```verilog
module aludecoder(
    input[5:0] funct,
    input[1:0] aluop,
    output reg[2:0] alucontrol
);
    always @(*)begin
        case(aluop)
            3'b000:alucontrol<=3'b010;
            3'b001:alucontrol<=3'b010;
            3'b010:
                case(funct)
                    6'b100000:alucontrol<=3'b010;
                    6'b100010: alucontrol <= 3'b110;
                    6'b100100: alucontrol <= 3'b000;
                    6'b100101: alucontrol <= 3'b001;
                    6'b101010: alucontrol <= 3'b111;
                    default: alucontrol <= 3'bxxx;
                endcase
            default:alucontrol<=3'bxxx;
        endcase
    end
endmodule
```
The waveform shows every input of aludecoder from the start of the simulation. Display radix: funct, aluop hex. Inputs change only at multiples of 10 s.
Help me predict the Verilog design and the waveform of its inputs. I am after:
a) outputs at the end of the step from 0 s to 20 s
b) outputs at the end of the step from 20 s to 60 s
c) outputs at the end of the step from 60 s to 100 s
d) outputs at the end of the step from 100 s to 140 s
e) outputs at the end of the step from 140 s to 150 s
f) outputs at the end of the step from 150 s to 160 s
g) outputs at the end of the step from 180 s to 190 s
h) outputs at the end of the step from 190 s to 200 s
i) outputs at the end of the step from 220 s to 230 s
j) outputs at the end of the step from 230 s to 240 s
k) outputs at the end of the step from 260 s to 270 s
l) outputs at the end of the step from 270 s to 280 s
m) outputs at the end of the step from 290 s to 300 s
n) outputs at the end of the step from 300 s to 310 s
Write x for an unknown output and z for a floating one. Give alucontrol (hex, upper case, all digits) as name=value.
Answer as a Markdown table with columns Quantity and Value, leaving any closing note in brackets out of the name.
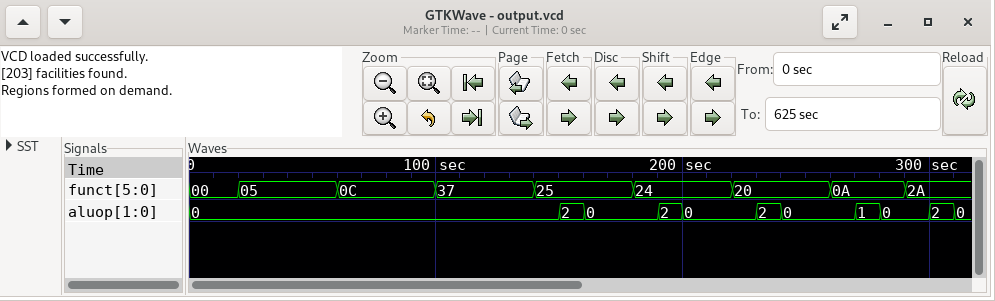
| Quantity | Value |
|---|---|
| outputs at the end of the step from 0 s to 20 s | alucontrol=2 |
| outputs at the end of the step from 20 s to 60 s | alucontrol=2 |
| outputs at the end of the step from 60 s to 100 s | alucontrol=2 |
| outputs at the end of the step from 100 s to 140 s | alucontrol=2 |
| outputs at the end of the step from 140 s to 150 s | alucontrol=2 |
| outputs at the end of the step from 150 s to 160 s | alucontrol=1 |
| outputs at the end of the step from 180 s to 190 s | alucontrol=2 |
| outputs at the end of the step from 190 s to 200 s | alucontrol=0 |
| outputs at the end of the step from 220 s to 230 s | alucontrol=2 |
| outputs at the end of the step from 230 s to 240 s | alucontrol=2 |
| outputs at the end of the step from 260 s to 270 s | alucontrol=2 |
| outputs at the end of the step from 270 s to 280 s | alucontrol=2 |
| outputs at the end of the step from 290 s to 300 s | alucontrol=2 |
| outputs at the end of the step from 300 s to 310 s | alucontrol=7 |
